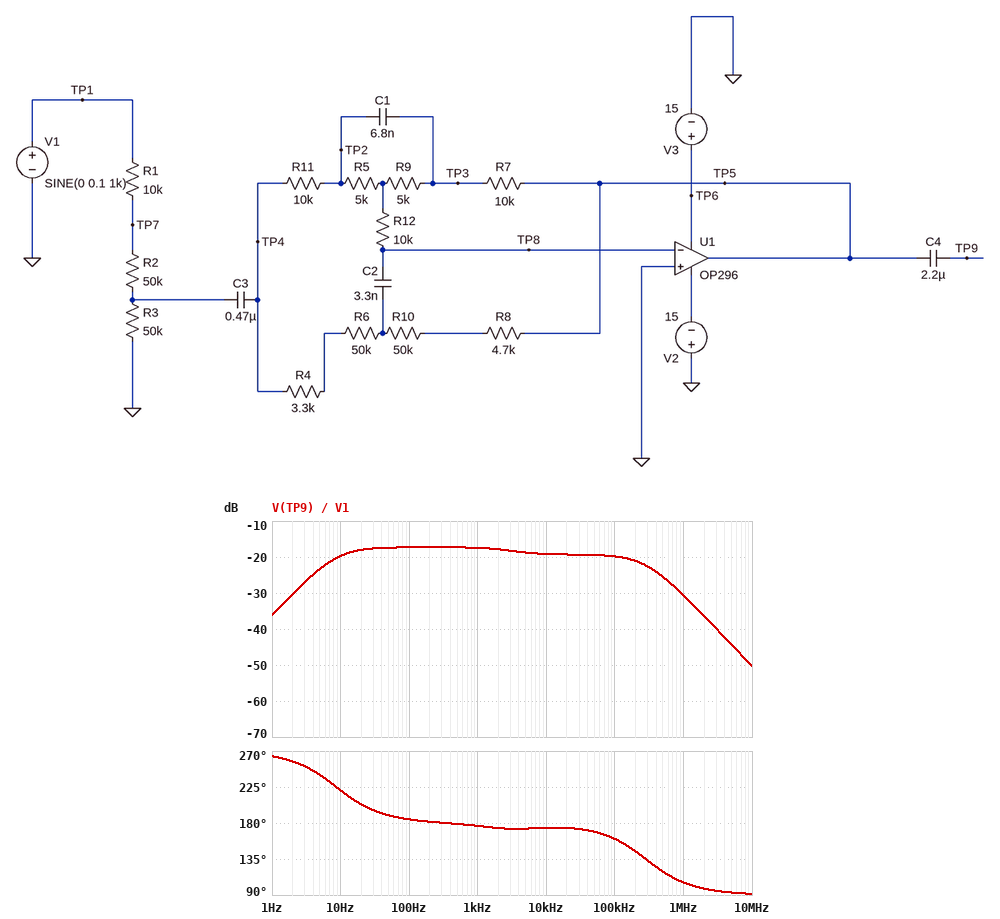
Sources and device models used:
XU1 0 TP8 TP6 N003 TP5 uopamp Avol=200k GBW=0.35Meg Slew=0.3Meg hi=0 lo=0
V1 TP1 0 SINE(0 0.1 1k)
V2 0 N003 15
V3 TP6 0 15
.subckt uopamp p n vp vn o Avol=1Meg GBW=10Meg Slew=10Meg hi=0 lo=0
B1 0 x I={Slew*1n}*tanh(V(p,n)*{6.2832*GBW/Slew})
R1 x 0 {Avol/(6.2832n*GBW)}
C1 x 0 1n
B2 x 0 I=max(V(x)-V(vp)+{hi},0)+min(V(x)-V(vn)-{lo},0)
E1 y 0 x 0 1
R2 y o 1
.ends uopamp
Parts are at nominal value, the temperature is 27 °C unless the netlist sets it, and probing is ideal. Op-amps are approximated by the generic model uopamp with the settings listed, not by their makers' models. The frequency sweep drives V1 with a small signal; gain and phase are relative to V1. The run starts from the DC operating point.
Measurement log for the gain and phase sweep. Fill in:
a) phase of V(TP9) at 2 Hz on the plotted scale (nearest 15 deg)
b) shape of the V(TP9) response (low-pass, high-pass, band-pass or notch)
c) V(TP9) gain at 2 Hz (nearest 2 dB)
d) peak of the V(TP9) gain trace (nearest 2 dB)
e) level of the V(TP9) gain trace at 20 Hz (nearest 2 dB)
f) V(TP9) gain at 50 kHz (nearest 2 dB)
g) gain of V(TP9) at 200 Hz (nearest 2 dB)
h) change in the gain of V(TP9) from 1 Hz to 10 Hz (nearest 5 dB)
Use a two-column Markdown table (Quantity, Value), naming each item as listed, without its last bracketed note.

| Quantity | Value |
|---|---|
| phase of V(TP9) at 2 Hz on the plotted scale | 255 deg |
| shape of the V(TP9) response | band-pass |
| V(TP9) gain at 2 Hz | -30 dB |
| peak of the V(TP9) gain trace | -18 dB |
| level of the V(TP9) gain trace at 20 Hz | -18 dB |
| V(TP9) gain at 50 kHz | -20 dB |
| gain of V(TP9) at 200 Hz | -18 dB |
| change in the gain of V(TP9) from 1 Hz to 10 Hz | 15 dB |
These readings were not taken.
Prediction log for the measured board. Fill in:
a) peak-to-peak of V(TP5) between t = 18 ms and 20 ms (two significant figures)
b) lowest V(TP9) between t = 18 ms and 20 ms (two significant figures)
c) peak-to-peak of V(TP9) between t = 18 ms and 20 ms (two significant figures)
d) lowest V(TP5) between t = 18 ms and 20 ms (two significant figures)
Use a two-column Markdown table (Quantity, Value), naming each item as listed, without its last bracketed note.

| Quantity | Value |
|---|---|
| peak-to-peak of V(TP5) between t = 18 ms and 20 ms | 27 mV |
| lowest V(TP9) between t = 18 ms and 20 ms | -13 mV |
| peak-to-peak of V(TP9) between t = 18 ms and 20 ms | 27 mV |
| lowest V(TP5) between t = 18 ms and 20 ms | -13 mV |
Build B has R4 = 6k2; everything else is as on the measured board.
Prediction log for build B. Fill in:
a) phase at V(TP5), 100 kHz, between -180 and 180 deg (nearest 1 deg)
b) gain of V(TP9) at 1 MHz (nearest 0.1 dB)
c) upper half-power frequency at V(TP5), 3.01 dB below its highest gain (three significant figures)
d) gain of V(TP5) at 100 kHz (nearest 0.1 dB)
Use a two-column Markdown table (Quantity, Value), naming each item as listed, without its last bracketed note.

| Quantity | Value |
|---|---|
| phase at V(TP5), 100 kHz, between -180 and 180 deg | 160 deg |
| gain of V(TP9) at 1 MHz | -30.7 dB |
| upper half-power frequency at V(TP5), 3.01 dB below its highest gain | 133 kHz |
| gain of V(TP5) at 100 kHz | -19.9 dB |
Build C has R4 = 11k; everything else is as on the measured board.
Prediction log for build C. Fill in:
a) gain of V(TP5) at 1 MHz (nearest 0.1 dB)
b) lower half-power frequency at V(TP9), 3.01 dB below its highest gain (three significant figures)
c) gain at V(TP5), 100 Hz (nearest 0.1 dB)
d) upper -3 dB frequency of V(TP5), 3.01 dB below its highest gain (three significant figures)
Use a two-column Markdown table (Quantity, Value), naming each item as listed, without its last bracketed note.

| Quantity | Value |
|---|---|
| gain of V(TP5) at 1 MHz | -30.8 dB |
| lower half-power frequency at V(TP9), 3.01 dB below its highest gain | 8.59 Hz |
| gain at V(TP5), 100 Hz | -17.2 dB |
| upper -3 dB frequency of V(TP5), 3.01 dB below its highest gain | 118 kHz |
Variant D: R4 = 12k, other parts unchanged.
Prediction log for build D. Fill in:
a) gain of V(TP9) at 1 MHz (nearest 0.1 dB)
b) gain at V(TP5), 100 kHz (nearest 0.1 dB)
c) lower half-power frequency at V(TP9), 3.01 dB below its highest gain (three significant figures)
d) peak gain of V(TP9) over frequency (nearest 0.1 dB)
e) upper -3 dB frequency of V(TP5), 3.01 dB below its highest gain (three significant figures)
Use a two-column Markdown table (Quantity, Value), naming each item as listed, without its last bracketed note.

| Quantity | Value |
|---|---|
| gain of V(TP9) at 1 MHz | -30.8 dB |
| gain at V(TP5), 100 kHz | -20.1 dB |
| lower half-power frequency at V(TP9), 3.01 dB below its highest gain | 8.59 Hz |
| peak gain of V(TP9) over frequency | -17.2 dB |
| upper -3 dB frequency of V(TP5), 3.01 dB below its highest gain | 115 kHz |
